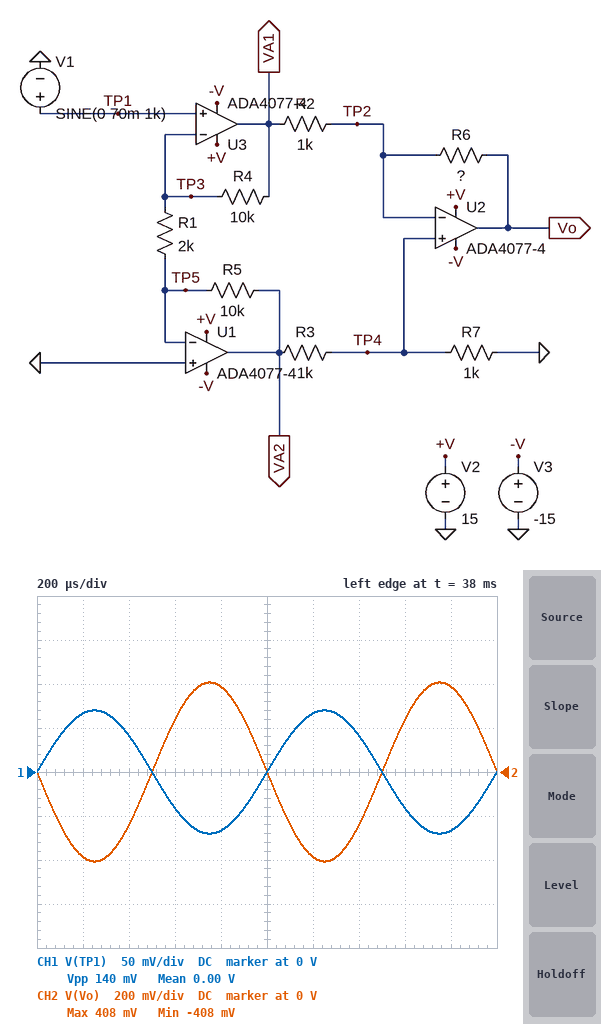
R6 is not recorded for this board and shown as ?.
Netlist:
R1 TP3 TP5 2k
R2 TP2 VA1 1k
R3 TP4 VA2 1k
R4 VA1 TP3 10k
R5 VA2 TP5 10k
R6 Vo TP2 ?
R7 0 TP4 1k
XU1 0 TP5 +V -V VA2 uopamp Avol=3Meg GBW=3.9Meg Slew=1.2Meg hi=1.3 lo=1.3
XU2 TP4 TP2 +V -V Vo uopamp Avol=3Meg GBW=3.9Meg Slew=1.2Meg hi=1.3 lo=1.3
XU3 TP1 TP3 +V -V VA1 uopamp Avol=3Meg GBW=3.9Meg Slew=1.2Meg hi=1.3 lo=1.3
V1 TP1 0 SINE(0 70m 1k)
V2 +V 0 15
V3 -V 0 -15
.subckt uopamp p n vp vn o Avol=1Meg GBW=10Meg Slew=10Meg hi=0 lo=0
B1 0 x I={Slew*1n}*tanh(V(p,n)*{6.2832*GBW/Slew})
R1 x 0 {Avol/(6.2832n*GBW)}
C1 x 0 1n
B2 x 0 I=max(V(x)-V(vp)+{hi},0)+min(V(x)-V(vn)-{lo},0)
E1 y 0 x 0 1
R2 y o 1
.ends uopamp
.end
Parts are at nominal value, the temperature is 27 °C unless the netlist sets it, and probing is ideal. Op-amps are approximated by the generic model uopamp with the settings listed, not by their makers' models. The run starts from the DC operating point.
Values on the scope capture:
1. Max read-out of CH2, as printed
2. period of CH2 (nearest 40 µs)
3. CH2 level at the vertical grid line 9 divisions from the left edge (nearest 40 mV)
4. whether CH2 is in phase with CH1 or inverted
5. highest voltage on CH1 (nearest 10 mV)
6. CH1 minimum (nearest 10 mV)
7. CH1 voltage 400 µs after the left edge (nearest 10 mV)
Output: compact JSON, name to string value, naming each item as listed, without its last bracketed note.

{"Max read-out of CH2, as printed": "408 mV", "period of CH2": "1.00 ms", "CH2 level at the vertical grid line 9 divisions from the left edge": "400 mV", "whether CH2 is in phase with CH1 or inverted": "inverted", "highest voltage on CH1": "70 mV", "CH1 minimum": "-70 mV", "CH1 voltage 400 µs after the left edge": "40 mV"}
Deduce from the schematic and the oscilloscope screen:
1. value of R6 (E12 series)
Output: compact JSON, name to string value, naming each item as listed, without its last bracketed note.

{"value of R6": "390 Ω"}
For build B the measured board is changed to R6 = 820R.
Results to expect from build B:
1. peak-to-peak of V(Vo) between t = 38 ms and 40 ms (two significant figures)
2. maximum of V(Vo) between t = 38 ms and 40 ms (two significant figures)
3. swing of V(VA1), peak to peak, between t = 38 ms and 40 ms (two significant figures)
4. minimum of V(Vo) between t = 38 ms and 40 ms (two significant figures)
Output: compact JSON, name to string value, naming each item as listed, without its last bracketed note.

{"peak-to-peak of V(Vo) between t = 38 ms and 40 ms": "1.3 V", "maximum of V(Vo) between t = 38 ms and 40 ms": "660 mV", "swing of V(VA1), peak to peak, between t = 38 ms and 40 ms": "840 mV", "minimum of V(Vo) between t = 38 ms and 40 ms": "-660 mV"}
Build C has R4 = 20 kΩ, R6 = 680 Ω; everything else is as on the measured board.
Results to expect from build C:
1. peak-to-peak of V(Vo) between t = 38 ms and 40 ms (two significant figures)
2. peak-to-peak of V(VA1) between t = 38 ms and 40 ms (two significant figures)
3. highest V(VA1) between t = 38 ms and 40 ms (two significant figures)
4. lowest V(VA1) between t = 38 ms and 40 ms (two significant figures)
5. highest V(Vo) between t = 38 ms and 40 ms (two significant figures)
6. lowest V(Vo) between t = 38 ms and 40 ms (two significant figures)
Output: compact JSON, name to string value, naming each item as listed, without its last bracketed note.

{"peak-to-peak of V(Vo) between t = 38 ms and 40 ms": "1.6 V", "peak-to-peak of V(VA1) between t = 38 ms and 40 ms": "1.5 V", "highest V(VA1) between t = 38 ms and 40 ms": "770 mV", "lowest V(VA1) between t = 38 ms and 40 ms": "-770 mV", "highest V(Vo) between t = 38 ms and 40 ms": "820 mV", "lowest V(Vo) between t = 38 ms and 40 ms": "-820 mV"}
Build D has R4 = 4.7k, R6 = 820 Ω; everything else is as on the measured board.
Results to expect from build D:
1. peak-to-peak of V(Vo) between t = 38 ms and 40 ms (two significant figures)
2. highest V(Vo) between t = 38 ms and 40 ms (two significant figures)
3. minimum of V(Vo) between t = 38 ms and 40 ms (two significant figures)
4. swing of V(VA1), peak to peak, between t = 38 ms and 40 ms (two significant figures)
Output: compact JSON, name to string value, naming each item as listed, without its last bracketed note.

{"peak-to-peak of V(Vo) between t = 38 ms and 40 ms": "1.0 V", "highest V(Vo) between t = 38 ms and 40 ms": "510 mV", "minimum of V(Vo) between t = 38 ms and 40 ms": "-510 mV", "swing of V(VA1), peak to peak, between t = 38 ms and 40 ms": "470 mV"}
